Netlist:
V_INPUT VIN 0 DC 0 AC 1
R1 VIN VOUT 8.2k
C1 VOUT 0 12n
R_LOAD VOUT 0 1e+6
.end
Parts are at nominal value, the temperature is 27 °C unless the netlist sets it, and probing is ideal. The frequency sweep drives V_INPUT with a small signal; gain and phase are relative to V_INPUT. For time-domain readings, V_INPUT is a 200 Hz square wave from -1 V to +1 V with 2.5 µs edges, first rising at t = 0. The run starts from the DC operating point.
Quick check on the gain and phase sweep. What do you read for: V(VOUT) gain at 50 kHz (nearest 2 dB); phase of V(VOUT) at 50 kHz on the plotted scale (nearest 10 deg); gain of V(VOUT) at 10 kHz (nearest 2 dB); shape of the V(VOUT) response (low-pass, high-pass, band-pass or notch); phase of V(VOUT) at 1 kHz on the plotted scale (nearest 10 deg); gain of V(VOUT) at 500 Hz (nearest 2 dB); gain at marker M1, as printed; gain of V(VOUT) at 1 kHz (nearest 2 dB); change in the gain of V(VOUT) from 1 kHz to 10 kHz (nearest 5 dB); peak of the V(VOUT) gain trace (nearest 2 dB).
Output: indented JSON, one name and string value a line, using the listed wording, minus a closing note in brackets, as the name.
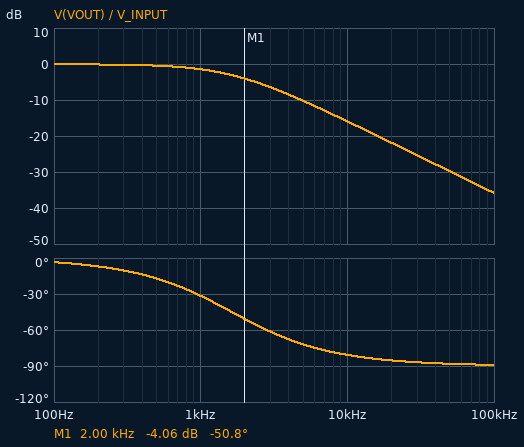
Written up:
{
  "V(VOUT) gain at 50 kHz": "-30 dB",
  "phase of V(VOUT) at 50 kHz on the plotted scale": "-90 deg",
  "gain of V(VOUT) at 10 kHz": "-16 dB",
  "shape of the V(VOUT) response": "low-pass",
  "phase of V(VOUT) at 1 kHz on the plotted scale": "-30 deg",
  "gain of V(VOUT) at 500 Hz": "0 dB",
  "gain at marker M1, as printed": "-4.06 dB",
  "gain of V(VOUT) at 1 kHz": "-2 dB",
  "change in the gain of V(VOUT) from 1 kHz to 10 kHz": "-15 dB",
  "peak of the V(VOUT) gain trace": "0 dB"
}
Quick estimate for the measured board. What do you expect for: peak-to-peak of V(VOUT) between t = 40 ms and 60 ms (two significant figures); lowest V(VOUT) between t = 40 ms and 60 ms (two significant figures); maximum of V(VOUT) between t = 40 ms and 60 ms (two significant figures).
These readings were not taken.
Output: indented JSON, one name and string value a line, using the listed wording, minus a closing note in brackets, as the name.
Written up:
{
  "peak-to-peak of V(VOUT) between t = 40 ms and 60 ms": "2.0 V",
  "lowest V(VOUT) between t = 40 ms and 60 ms": "-990 mV",
  "maximum of V(VOUT) between t = 40 ms and 60 ms": "990 mV"
}
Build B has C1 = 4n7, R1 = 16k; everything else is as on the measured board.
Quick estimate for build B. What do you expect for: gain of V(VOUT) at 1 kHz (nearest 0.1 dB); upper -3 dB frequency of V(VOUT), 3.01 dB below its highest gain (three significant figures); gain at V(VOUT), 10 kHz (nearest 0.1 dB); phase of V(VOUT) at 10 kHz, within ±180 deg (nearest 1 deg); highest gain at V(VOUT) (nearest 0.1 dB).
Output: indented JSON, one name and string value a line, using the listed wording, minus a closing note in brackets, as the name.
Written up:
{
  "gain of V(VOUT) at 1 kHz": "-1.0 dB",
  "upper -3 dB frequency of V(VOUT), 3.01 dB below its highest gain": "2.15 kHz",
  "gain at V(VOUT), 10 kHz": "-13.7 dB",
  "phase of V(VOUT) at 10 kHz, within ±180 deg": "-78 deg",
  "highest gain at V(VOUT)": "-0.1 dB"
}
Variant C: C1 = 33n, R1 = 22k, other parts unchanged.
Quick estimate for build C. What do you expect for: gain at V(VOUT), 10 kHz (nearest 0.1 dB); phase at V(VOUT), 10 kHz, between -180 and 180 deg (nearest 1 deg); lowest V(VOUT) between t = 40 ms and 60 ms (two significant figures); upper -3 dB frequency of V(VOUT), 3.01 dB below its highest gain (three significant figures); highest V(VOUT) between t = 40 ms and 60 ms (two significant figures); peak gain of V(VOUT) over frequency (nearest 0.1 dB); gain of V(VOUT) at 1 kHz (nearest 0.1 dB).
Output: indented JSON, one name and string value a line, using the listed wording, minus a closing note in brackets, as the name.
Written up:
{
  "gain at V(VOUT), 10 kHz": "-33.2 dB",
  "phase at V(VOUT), 10 kHz, between -180 and 180 deg": "-89 deg",
  "lowest V(VOUT) between t = 40 ms and 60 ms": "-920 mV",
  "upper -3 dB frequency of V(VOUT), 3.01 dB below its highest gain": "224 Hz",
  "highest V(VOUT) between t = 40 ms and 60 ms": "920 mV",
  "peak gain of V(VOUT) over frequency": "-0.2 dB",
  "gain of V(VOUT) at 1 kHz": "-13.4 dB"
}
